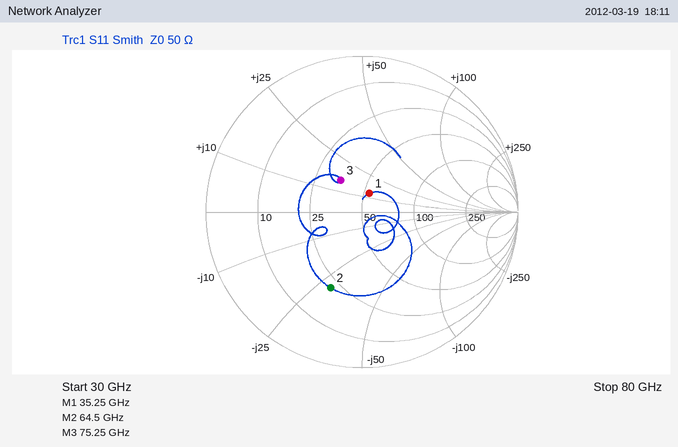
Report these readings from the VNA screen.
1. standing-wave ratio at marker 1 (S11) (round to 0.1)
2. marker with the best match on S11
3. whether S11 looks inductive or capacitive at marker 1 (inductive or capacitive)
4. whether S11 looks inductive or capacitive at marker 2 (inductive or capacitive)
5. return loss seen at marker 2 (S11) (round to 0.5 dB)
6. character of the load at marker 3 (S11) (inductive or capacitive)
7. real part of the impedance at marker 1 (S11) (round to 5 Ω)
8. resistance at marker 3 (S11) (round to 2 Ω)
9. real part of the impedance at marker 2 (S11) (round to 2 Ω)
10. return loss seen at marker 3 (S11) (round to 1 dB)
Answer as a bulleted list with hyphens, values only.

- 1.3
- marker 1
- inductive
- capacitive
- 5.5 dB
- inductive
- 55 Ω
- 36 Ω
- 22 Ω
- 12 dB
